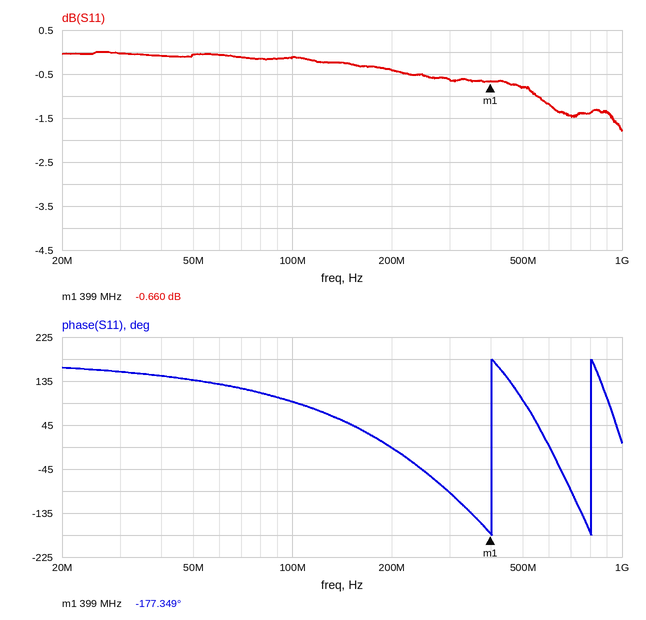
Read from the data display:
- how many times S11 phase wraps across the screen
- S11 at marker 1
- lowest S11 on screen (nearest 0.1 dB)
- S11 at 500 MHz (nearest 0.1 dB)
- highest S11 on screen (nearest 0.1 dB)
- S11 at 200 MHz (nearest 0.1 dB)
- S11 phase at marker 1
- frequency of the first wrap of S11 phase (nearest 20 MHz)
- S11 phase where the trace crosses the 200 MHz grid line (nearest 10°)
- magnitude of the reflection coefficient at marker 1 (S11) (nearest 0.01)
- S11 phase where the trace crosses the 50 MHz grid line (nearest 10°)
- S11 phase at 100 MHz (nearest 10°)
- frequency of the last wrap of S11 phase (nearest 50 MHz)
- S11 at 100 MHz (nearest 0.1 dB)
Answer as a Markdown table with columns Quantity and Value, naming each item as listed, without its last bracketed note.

| Quantity | Value |
|---|---|
| how many times S11 phase wraps across the screen | 2 |
| S11 at marker 1 | -0.660 dB |
| lowest S11 on screen | -1.8 dB |
| S11 at 500 MHz | -0.8 dB |
| highest S11 on screen | 0.0 dB |
| S11 at 200 MHz | -0.4 dB |
| S11 phase at marker 1 | -177.349° |
| frequency of the first wrap of S11 phase | 400 MHz |
| S11 phase where the trace crosses the 200 MHz grid line | 0° |
| magnitude of the reflection coefficient at marker 1 (S11) | 0.93 |
| S11 phase where the trace crosses the 50 MHz grid line | 140° |
| S11 phase at 100 MHz | 90° |
| frequency of the last wrap of S11 phase | 800 MHz |
| S11 at 100 MHz | -0.1 dB |
